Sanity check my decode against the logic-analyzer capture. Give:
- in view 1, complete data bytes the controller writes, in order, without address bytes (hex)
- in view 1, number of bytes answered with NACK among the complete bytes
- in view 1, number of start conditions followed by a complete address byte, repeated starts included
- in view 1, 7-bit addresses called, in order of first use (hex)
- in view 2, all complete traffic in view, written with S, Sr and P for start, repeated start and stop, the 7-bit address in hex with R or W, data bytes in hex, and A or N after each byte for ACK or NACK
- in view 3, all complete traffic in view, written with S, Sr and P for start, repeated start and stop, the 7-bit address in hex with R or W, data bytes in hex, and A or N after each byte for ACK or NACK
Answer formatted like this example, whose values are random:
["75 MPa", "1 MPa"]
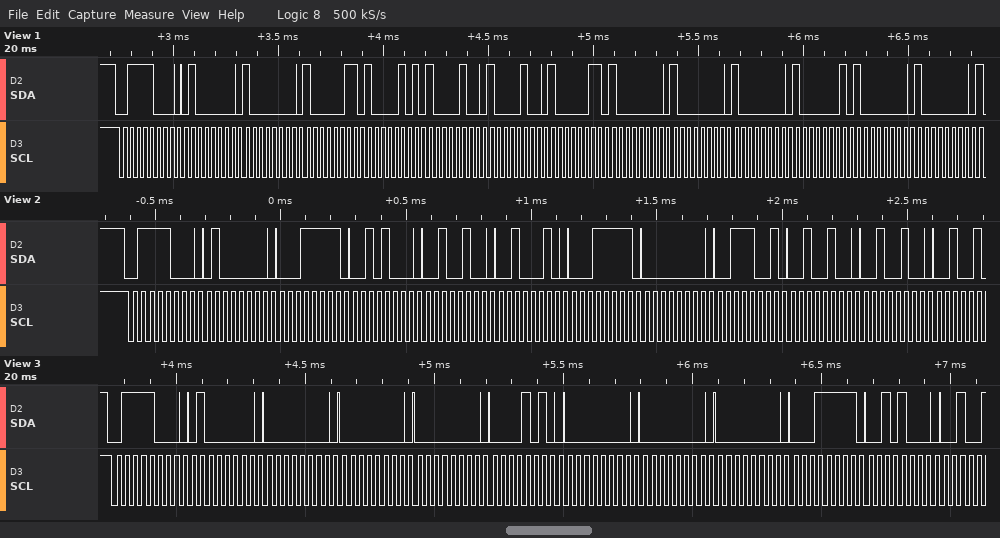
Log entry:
["40 80 83 85 84 84 83 80 80 80 81 80 80", "0", "1", "0x3C", "S 3CW A 40 A 1F A 28 A 24 A 22 A 1F A 00 A 39 A 24 A 24 A", "S 3CW A 40 A 00 A 00 A 00 A 0A A 00 A 00 A 00 A 1F A 28 A"]
